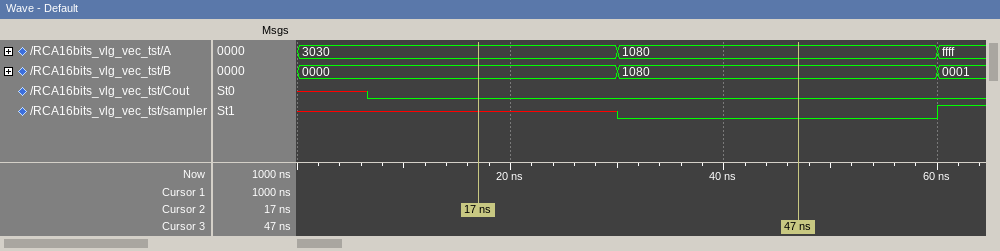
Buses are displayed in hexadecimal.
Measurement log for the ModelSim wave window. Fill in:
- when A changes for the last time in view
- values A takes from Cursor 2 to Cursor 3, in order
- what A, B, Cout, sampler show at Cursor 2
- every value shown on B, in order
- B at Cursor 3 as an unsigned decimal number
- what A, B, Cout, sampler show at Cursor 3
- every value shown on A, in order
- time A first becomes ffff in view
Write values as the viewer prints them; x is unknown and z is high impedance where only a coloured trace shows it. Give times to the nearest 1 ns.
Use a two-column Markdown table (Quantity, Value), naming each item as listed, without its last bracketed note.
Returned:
| Quantity | Value |
|---|---|
| when A changes for the last time in view | 60 ns |
| values A takes from Cursor 2 to Cursor 3, in order | 3030, 1080 |
| what A, B, Cout, sampler show at Cursor 2 | A=3030, B=0000, Cout=0, sampler=x |
| every value shown on B, in order | 0000, 1080, 0001 |
| B at Cursor 3 as an unsigned decimal number | 4224 |
| what A, B, Cout, sampler show at Cursor 3 | A=1080, B=1080, Cout=0, sampler=0 |
| every value shown on A, in order | 3030, 1080, ffff |
| time A first becomes ffff in view | 60 ns |
